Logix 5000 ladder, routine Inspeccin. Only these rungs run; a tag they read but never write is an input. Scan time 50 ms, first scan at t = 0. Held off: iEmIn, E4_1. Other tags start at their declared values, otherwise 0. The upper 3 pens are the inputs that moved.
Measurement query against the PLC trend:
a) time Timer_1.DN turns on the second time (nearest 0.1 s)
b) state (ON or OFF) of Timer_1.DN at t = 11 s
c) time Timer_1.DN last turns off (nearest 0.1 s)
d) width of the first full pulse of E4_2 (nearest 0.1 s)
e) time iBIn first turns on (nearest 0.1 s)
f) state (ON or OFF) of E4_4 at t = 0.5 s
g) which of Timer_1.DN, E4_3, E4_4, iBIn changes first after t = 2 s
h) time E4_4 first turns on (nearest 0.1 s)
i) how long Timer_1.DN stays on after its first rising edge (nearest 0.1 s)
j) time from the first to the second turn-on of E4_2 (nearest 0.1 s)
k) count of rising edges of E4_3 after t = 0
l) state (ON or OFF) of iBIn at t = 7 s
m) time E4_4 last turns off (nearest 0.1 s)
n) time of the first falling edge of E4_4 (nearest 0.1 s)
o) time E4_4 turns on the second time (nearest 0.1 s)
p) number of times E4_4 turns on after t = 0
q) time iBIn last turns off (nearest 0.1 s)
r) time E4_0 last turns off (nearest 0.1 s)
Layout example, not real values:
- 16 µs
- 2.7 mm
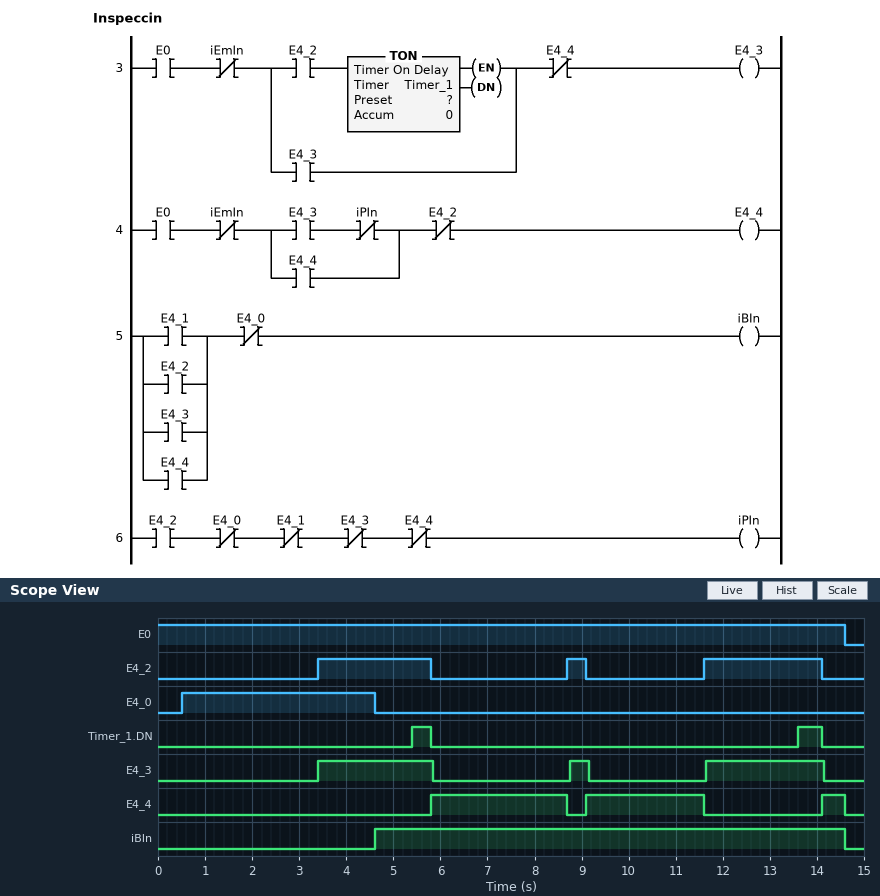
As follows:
- 13.6 s
- OFF
- 14.1 s
- 2.4 s
- 4.6 s
- OFF
- E4_3
- 5.8 s
- 0.4 s
- 5.3 s
- 3
- ON
- 14.6 s
- 8.7 s
- 9.1 s
- 3
- 14.6 s
- 4.6 s
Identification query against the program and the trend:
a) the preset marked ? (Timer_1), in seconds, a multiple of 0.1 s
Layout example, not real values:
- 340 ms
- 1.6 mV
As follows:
- 2.0 s
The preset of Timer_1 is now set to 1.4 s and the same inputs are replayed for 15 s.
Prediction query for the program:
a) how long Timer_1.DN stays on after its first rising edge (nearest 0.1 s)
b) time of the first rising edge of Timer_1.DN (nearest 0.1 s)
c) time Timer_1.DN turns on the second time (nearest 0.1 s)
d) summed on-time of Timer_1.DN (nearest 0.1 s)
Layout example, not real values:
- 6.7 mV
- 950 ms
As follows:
- 1.0 s
- 4.8 s
- 13.0 s
- 2.1 s
